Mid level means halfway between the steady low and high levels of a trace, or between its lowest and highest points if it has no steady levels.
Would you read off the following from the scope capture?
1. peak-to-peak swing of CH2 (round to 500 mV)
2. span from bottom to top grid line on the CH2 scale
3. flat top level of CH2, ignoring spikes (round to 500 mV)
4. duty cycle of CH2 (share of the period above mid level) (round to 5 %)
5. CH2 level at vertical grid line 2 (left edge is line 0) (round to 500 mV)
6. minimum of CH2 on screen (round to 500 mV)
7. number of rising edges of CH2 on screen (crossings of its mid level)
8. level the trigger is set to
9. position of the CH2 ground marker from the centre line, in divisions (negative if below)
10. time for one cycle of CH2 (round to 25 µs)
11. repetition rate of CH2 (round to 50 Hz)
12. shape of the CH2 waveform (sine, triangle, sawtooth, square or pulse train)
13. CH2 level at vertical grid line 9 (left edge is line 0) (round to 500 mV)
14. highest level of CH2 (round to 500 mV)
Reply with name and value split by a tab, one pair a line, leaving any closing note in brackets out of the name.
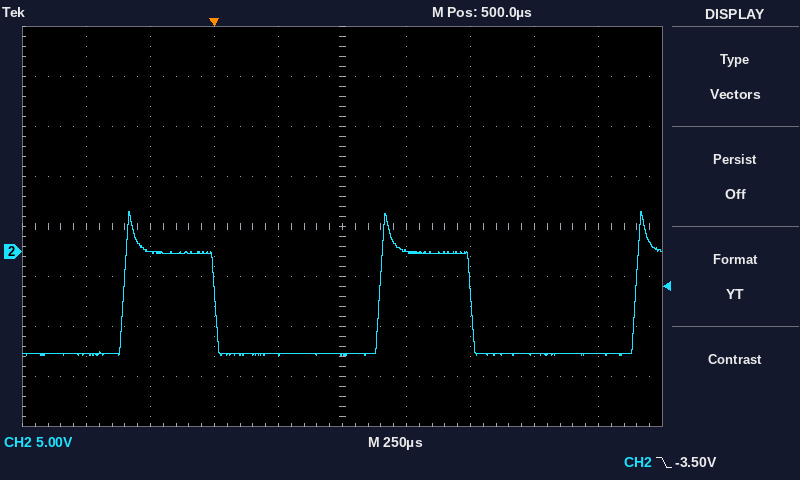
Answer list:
peak-to-peak swing of CH2	14.5 V
span from bottom to top grid line on the CH2 scale	40 V
flat top level of CH2, ignoring spikes	0.0 V
duty cycle of CH2 (share of the period above mid level)	35 %
CH2 level at vertical grid line 2 (left edge is line 0)	0.0 V
minimum of CH2 on screen	-10.5 V
number of rising edges of CH2 on screen	3
level the trigger is set to	-3.50 V
position of the CH2 ground marker from the centre line, in divisions	-0.5 div
time for one cycle of CH2	1.000 ms
repetition rate of CH2	1.00 kHz
shape of the CH2 waveform	pulse train
CH2 level at vertical grid line 9 (left edge is line 0)	-10.0 V
highest level of CH2	4.0 V
